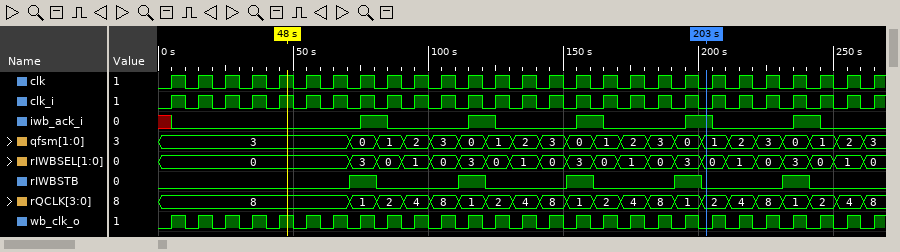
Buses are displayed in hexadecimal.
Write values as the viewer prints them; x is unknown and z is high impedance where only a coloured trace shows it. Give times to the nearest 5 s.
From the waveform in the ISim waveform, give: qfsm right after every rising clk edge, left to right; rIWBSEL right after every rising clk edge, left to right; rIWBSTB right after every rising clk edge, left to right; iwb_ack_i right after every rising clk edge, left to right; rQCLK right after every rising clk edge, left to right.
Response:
3, 3, 3, 3, 3, 3, 3, 0, 1, 2, 3, 0, 1, 2, 3, 0, 1, 2, 3, 0, 1, 2, 3, 0, 1, 2, 3
0, 0, 0, 0, 0, 0, 0, 3, 0, 1, 0, 3, 0, 1, 0, 3, 0, 1, 0, 3, 0, 1, 0, 3, 0, 1, 0
0 0 0 0 0 0 0 1 0 0 0 1 0 0 0 1 0 0 0 1 0 0 0 1 0 0 0
0 0 0 0 0 0 0 1 0 0 0 1 0 0 0 1 0 0 0 1 0 0 0 1 0 0 0
8, 8, 8, 8, 8, 8, 8, 1, 2, 4, 8, 1, 2, 4, 8, 1, 2, 4, 8, 1, 2, 4, 8, 1, 2, 4, 8
